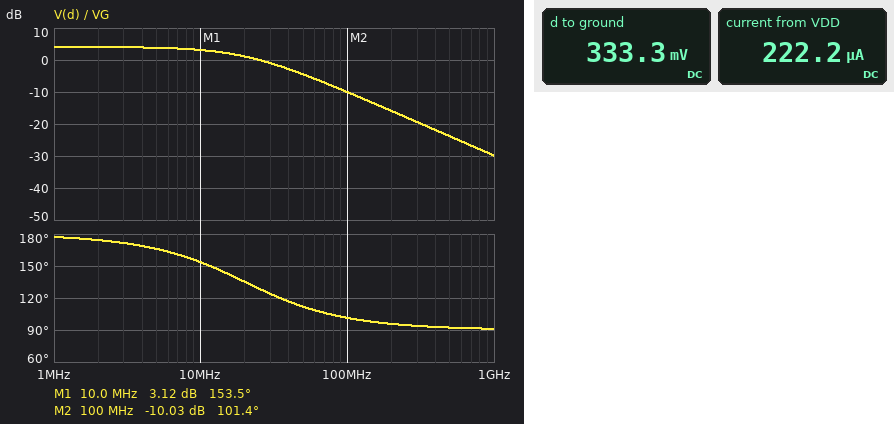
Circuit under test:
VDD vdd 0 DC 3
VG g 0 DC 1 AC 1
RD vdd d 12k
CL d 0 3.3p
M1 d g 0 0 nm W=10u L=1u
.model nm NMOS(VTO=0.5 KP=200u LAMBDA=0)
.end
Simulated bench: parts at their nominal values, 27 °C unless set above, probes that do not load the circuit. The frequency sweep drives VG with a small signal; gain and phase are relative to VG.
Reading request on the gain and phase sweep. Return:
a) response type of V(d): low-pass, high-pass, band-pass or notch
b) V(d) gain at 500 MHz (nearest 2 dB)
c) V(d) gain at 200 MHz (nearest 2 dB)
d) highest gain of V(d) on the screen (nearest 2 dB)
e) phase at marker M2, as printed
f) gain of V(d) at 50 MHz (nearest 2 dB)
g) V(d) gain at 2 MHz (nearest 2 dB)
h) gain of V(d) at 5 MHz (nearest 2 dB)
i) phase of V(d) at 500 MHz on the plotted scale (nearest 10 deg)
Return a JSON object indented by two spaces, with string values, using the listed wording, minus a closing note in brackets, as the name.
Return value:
{
  "response type of V(d): low-pass, high-pass, band-pass or notch": "low-pass",
  "V(d) gain at 500 MHz": "-24 dB",
  "V(d) gain at 200 MHz": "-16 dB",
  "highest gain of V(d) on the screen": "4 dB",
  "phase at marker M2, as printed": "101.4 deg",
  "gain of V(d) at 50 MHz": "-4 dB",
  "V(d) gain at 2 MHz": "4 dB",
  "gain of V(d) at 5 MHz": "4 dB",
  "phase of V(d) at 500 MHz on the plotted scale": "90 deg"
}
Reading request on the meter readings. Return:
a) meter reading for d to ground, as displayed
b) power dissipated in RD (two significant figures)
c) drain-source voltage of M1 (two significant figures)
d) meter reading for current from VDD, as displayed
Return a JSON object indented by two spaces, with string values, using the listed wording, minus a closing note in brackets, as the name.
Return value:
{
  "meter reading for d to ground, as displayed": "333.3 mV",
  "power dissipated in RD": "590 µW",
  "drain-source voltage of M1": "330 mV",
  "meter reading for current from VDD, as displayed": "222.2 µA"
}
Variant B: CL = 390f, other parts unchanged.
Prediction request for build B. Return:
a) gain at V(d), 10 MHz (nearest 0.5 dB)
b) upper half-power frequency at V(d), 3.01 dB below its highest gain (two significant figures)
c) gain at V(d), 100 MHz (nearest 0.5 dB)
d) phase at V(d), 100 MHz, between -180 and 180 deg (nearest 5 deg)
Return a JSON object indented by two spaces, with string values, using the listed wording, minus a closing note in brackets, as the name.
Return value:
{
  "gain at V(d), 10 MHz": "4.0 dB",
  "upper half-power frequency at V(d), 3.01 dB below its highest gain": "170 MHz",
  "gain at V(d), 100 MHz": "3.0 dB",
  "phase at V(d), 100 MHz, between -180 and 180 deg": "150 deg"
}
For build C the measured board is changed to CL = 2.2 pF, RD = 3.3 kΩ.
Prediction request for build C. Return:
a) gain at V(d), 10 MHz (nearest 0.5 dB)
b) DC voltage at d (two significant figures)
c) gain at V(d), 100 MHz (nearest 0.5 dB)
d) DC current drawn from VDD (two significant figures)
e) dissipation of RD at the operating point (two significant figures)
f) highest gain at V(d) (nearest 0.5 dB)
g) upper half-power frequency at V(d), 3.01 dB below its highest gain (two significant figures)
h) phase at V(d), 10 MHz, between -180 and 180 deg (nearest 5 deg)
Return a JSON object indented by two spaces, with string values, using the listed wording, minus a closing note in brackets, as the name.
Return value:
{
  "gain at V(d), 10 MHz": "9.5 dB",
  "DC voltage at d": "2.2 V",
  "gain at V(d), 100 MHz": "-3.0 dB",
  "DC current drawn from VDD": "250 µA",
  "dissipation of RD at the operating point": "210 µW",
  "highest gain at V(d)": "10.5 dB",
  "upper half-power frequency at V(d), 3.01 dB below its highest gain": "22 MHz",
  "phase at V(d), 10 MHz, between -180 and 180 deg": "155 deg"
}
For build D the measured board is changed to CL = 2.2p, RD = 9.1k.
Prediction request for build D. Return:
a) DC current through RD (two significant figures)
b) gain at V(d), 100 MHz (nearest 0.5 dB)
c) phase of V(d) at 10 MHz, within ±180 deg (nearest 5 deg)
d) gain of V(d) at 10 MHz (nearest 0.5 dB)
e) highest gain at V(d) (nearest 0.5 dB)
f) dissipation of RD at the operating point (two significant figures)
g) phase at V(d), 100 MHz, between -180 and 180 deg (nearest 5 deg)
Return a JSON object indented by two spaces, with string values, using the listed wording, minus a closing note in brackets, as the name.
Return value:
{
  "DC current through RD": "250 µA",
  "gain at V(d), 100 MHz": "-3.0 dB",
  "phase of V(d) at 10 MHz, within ±180 deg": "130 deg",
  "gain of V(d) at 10 MHz": "15.0 dB",
  "highest gain at V(d)": "19.0 dB",
  "dissipation of RD at the operating point": "570 µW",
  "phase at V(d), 100 MHz, between -180 and 180 deg": "95 deg"
}
